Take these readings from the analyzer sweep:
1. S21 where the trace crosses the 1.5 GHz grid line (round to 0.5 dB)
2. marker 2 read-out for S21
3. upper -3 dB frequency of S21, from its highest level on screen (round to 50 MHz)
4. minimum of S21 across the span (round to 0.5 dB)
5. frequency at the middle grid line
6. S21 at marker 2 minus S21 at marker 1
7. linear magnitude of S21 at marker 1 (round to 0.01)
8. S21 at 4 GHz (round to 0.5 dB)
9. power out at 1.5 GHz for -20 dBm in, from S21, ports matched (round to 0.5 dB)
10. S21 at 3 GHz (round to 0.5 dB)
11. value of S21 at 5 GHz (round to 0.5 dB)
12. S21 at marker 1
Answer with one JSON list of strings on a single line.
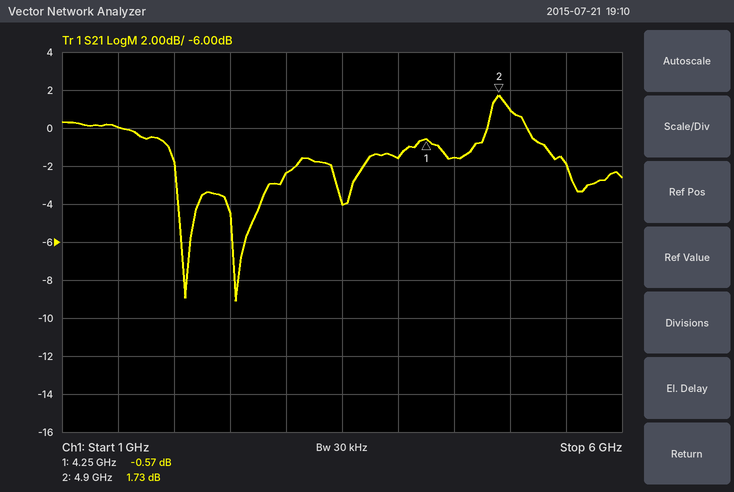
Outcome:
["0.0 dB", "1.73 dB", "5.35 GHz", "-9.0 dB", "3.5 GHz", "2.30 dB", "0.94", "-1.5 dB", "-20.0 dBm", "-2.5 dB", "1.0 dB", "-0.57 dB"]
